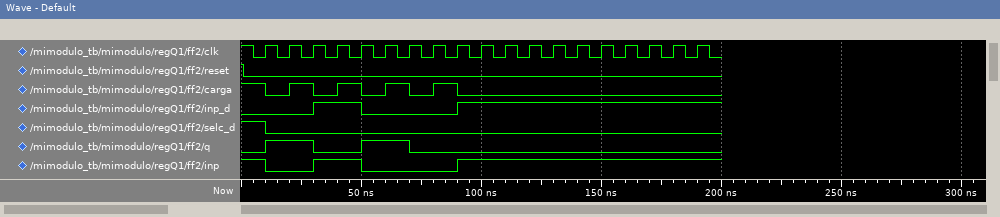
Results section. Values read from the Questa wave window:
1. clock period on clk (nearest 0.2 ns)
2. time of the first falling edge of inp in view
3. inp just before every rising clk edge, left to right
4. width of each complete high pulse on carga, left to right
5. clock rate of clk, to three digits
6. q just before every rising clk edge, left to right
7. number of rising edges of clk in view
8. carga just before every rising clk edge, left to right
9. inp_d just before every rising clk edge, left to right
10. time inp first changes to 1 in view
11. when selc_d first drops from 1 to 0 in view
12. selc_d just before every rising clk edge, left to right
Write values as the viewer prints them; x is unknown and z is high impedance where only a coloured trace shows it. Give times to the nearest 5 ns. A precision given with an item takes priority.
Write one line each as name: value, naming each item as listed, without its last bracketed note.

clock period on clk: 10 ns
time of the first falling edge of inp in view: 10 ns
inp just before every rising clk edge, left to right: 1 0 0 1 1 0 0 0 0 1 1 1 1 1 1 1 1 1 1
width of each complete high pulse on carga, left to right: 10 ns, 10 ns, 10 ns, 10 ns
clock rate of clk, to three digits: 100 MHz
q just before every rising clk edge, left to right: 0 1 1 0 0 1 1 0 0 0 0 0 0 0 0 0 0 0 0
number of rising edges of clk in view: 19
carga just before every rising clk edge, left to right: 1 0 1 0 1 0 1 0 1 0 0 0 0 0 0 0 0 0 0
inp_d just before every rising clk edge, left to right: 0 0 0 1 1 0 0 0 0 1 1 1 1 1 1 1 1 1 1
time inp first changes to 1 in view: 30 ns
when selc_d first drops from 1 to 0 in view: 10 ns
selc_d just before every rising clk edge, left to right: 1 0 0 0 0 0 0 0 0 0 0 0 0 0 0 0 0 0 0
